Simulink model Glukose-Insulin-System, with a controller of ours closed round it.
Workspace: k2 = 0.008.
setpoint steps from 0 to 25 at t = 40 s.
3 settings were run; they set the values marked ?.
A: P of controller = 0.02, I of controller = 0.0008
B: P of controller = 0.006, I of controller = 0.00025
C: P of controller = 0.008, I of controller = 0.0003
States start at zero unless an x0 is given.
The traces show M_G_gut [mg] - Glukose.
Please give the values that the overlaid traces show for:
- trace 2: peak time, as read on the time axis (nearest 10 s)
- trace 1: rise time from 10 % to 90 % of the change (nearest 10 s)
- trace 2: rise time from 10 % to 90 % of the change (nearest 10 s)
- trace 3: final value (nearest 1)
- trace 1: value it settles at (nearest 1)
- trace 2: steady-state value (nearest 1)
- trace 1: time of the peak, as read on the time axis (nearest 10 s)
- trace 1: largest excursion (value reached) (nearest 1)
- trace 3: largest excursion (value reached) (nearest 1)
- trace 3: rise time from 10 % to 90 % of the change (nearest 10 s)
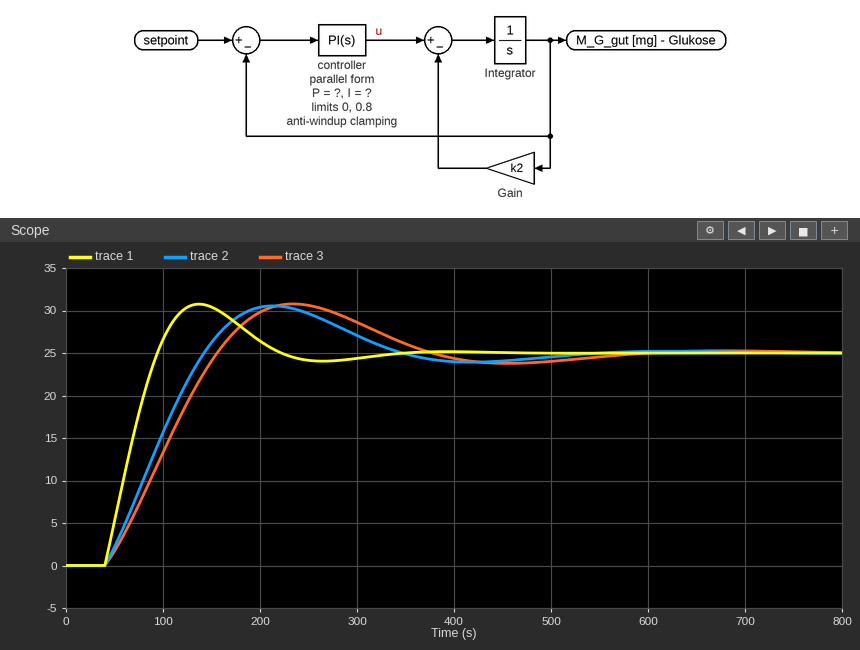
210 s
40 s
80 s
25
25
25
140 s
31
31
90 s
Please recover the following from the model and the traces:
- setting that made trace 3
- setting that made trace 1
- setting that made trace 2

B
A
C
